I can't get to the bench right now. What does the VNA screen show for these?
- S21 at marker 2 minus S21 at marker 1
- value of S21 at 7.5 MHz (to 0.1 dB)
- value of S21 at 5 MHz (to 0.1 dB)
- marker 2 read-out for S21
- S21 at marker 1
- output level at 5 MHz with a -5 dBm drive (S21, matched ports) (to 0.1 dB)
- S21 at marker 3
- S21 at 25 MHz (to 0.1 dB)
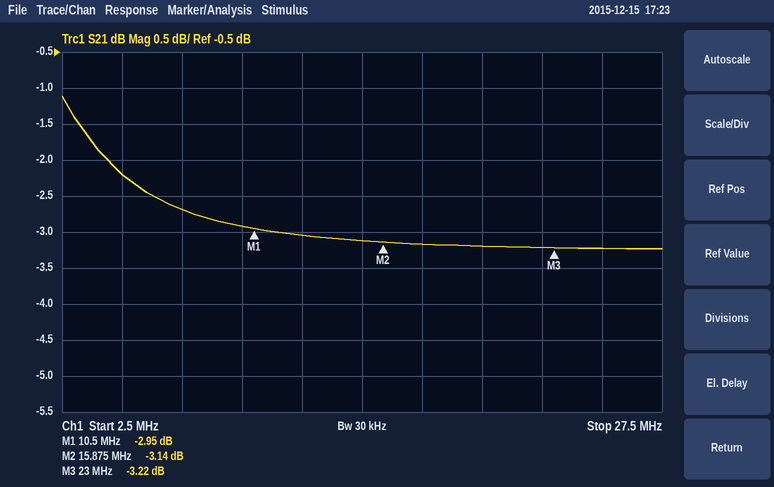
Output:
-0.19 dB
-2.7 dB
-2.2 dB
-3.14 dB
-2.95 dB
-7.2 dBm
-3.22 dB
-3.2 dB
